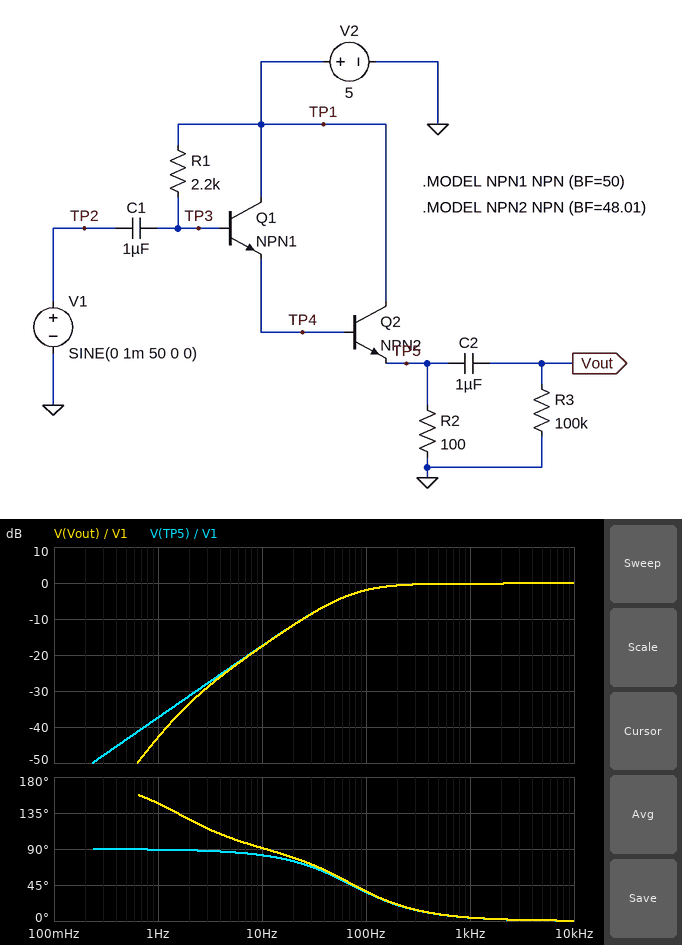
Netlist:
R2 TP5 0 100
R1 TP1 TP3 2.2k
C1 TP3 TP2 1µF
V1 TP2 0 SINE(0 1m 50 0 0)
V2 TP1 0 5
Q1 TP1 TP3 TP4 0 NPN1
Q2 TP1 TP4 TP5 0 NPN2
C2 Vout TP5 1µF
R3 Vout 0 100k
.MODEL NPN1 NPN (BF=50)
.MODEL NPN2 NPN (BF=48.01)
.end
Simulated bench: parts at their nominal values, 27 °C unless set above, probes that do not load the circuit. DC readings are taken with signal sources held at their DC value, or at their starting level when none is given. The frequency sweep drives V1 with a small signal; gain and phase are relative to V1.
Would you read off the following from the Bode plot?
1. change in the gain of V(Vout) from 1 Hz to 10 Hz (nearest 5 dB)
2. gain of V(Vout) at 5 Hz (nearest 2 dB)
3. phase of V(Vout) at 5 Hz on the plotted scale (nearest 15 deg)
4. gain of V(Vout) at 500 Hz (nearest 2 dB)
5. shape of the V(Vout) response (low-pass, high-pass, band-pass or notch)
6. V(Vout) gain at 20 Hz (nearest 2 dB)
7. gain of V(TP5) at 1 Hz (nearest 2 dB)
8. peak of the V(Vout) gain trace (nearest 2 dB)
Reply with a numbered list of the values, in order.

1. 25 dB
2. -24 dB
3. 105 deg
4. 0 dB
5. high-pass
6. -12 dB
7. -38 dB
8. 0 dB
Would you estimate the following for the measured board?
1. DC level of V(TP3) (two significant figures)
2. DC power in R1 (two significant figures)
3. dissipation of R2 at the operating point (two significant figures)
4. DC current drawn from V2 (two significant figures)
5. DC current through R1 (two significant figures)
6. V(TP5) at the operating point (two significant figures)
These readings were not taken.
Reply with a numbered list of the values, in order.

1. 5.0 V
2. 390 nW
3. 110 mW
4. 33 mA
5. 13 µA
6. 3.3 V
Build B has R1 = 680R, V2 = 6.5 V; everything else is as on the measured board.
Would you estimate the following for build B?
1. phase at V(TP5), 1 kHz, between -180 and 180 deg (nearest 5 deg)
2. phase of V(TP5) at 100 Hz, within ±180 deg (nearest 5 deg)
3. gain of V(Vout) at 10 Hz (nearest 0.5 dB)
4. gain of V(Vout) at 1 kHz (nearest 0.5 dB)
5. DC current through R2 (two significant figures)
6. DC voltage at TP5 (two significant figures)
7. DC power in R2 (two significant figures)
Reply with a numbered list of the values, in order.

1. 15 deg
2. 65 deg
3. -27.5 dB
4. -0.5 dB
5. 48 mA
6. 4.8 V
7. 230 mW
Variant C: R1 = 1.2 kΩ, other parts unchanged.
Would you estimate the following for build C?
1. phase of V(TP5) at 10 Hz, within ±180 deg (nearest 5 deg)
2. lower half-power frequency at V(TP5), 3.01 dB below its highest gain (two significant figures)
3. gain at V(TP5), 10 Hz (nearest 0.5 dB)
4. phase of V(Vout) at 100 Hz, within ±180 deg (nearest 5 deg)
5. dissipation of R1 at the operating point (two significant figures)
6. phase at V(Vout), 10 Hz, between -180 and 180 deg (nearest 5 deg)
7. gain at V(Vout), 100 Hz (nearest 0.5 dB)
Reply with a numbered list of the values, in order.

1. 85 deg
2. 130 Hz
3. -22.5 dB
4. 55 deg
5. 220 nW
6. 95 deg
7. -4.5 dB
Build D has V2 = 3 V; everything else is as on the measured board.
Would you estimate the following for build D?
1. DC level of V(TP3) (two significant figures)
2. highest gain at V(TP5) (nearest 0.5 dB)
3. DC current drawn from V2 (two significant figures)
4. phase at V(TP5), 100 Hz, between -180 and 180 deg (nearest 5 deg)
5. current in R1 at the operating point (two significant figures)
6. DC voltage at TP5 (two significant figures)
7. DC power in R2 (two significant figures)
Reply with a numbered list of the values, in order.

1. 3.0 V
2. -0.5 dB
3. 14 mA
4. 35 deg
5. 5.6 µA
6. 1.4 V
7. 20 mW
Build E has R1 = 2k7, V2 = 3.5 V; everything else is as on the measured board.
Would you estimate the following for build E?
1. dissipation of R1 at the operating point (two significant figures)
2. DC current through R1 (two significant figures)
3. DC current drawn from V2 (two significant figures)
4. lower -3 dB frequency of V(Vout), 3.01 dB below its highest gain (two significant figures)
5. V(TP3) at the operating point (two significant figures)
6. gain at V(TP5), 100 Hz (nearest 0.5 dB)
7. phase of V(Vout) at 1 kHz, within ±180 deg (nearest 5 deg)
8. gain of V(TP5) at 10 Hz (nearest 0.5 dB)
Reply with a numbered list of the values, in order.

1. 150 nW
2. 7.5 µA
3. 19 mA
4. 60 Hz
5. 3.5 V
6. -1.5 dB
7. 5 deg
8. -16.0 dB
